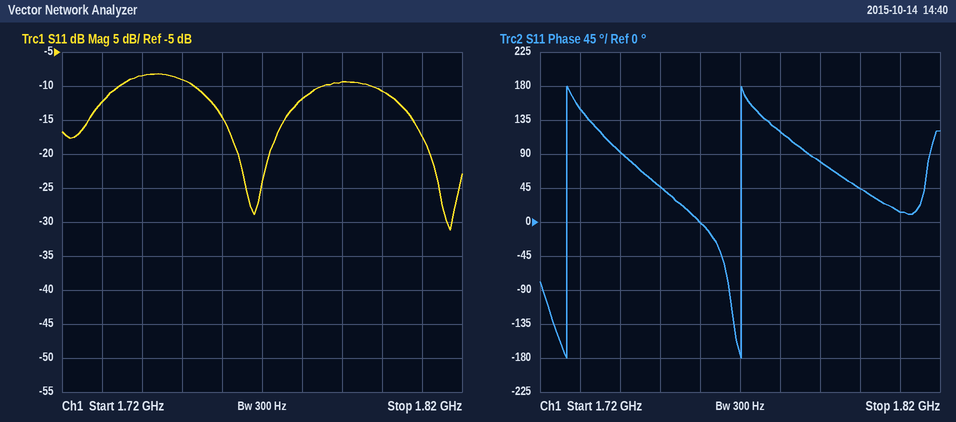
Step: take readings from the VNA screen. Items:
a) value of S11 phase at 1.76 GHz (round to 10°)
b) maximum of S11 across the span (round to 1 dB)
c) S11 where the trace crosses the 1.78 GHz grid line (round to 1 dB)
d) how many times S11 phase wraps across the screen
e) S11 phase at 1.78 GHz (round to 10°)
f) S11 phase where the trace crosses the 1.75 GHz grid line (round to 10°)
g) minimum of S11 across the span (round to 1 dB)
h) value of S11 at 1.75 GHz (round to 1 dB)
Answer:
0°
-8 dB
-12 dB
2
120°
50°
-31 dB
-9 dB
